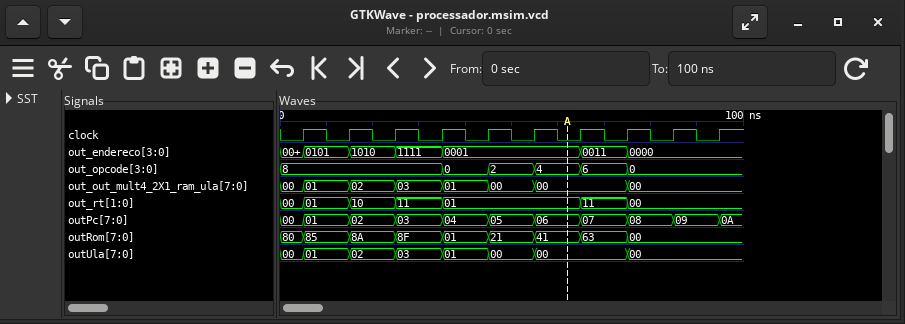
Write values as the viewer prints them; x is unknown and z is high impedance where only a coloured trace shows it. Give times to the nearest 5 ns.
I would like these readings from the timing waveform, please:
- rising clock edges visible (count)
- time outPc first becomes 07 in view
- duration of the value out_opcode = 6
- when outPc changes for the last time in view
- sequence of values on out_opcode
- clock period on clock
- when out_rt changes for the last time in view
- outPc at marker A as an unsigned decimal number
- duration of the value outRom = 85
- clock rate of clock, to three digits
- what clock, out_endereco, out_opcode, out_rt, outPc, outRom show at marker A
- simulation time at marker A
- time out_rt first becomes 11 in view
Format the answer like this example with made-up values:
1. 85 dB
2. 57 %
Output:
1. 10
2. 65 ns
3. 10 ns
4. 95 ns
5. 8, 0, 2, 4, 6, 0
6. 10 ns
7. 75 ns
8. 6
9. 10 ns
10. 100 MHz
11. clock=0, out_endereco=0001, out_opcode=4, out_rt=01, outPc=06, outRom=41
12. 60 ns
13. 25 ns
